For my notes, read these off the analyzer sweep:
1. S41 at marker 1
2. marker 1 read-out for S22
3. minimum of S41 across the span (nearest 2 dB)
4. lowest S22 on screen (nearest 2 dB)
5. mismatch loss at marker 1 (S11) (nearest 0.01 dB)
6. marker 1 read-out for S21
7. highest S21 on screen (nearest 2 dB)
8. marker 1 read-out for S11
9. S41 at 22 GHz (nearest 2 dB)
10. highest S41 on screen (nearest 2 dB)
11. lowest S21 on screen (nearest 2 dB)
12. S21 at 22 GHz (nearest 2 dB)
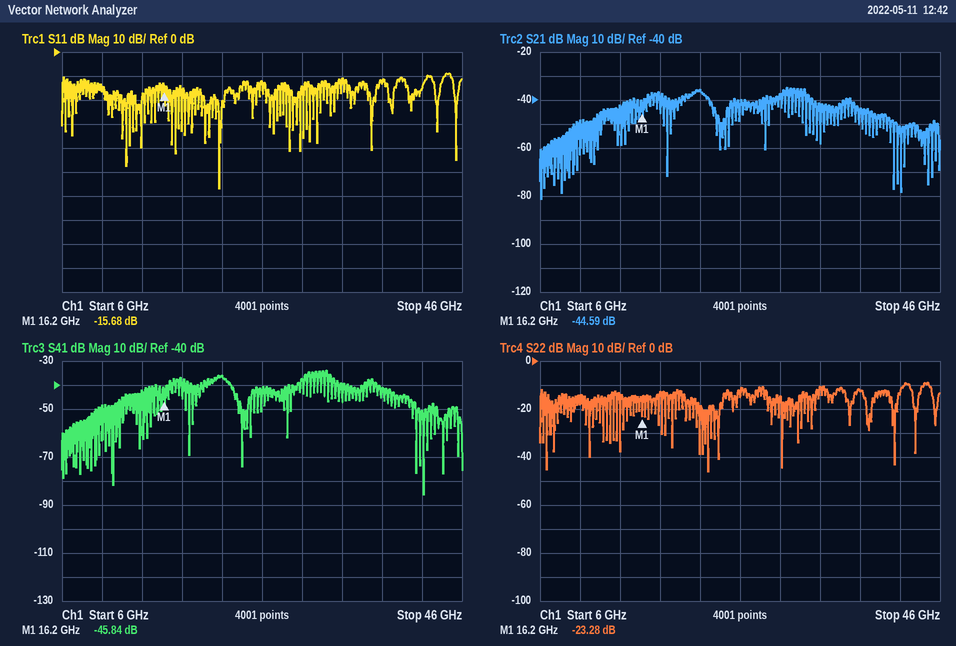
-45.84 dB
-23.28 dB
-86 dB
-46 dB
0.12 dB
-44.59 dB
-34 dB
-15.68 dB
-36 dB
-34 dB
-82 dB
-36 dB
